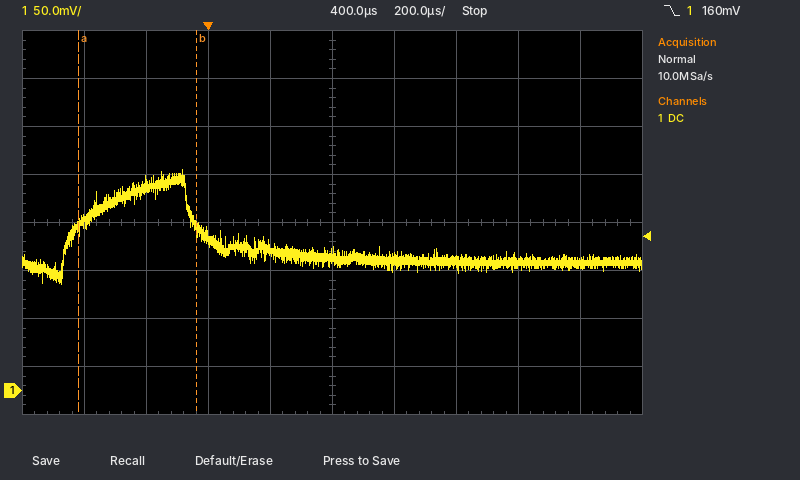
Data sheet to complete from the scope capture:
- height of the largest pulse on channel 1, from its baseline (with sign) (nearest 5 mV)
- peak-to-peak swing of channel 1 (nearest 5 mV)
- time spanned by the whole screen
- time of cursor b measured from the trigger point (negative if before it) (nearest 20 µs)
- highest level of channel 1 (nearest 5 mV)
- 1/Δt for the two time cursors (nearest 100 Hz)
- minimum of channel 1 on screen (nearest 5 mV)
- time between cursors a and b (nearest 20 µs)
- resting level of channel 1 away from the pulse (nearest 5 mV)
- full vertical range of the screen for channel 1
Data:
+95 mV
120 mV
2 ms
-40 µs
230 mV
2.6 kHz
110 mV
380 µs
135 mV
400 mV
